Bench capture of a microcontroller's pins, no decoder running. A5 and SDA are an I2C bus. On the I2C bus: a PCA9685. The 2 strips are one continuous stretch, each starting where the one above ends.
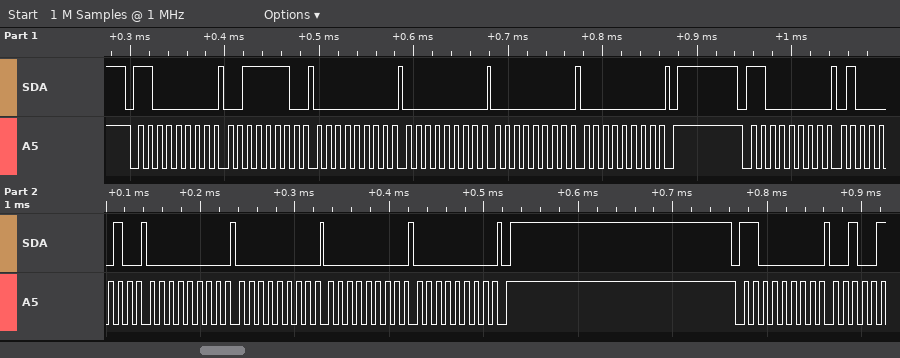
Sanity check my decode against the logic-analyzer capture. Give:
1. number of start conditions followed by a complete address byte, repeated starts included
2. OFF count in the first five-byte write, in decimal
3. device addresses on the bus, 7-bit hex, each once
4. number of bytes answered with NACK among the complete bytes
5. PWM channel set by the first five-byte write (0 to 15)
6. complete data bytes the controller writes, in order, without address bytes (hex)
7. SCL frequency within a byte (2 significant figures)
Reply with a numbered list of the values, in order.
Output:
1. 3
2. 0
3. 0x60
4. 0
5. 14
6. 3E 00 00 00 00 42 00 00 00 00
7. 100 kHz
